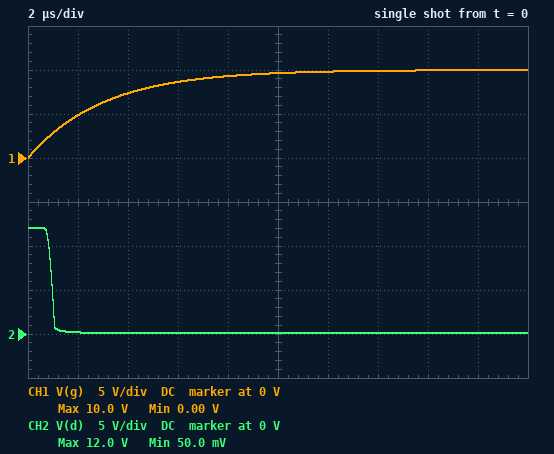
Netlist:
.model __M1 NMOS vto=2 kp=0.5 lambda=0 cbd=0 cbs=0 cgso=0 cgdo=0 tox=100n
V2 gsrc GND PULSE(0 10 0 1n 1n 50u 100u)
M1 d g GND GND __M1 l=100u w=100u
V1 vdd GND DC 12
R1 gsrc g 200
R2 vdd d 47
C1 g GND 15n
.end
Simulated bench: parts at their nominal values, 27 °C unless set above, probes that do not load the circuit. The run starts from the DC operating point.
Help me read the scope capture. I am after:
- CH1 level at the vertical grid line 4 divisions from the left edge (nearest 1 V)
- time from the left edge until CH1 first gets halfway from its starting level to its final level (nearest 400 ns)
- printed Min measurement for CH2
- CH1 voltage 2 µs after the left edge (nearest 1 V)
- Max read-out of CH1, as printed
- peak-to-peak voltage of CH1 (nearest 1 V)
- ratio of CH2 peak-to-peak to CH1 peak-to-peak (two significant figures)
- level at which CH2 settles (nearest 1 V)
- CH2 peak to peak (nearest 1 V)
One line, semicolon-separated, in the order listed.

9 V; 2.0 µs; 50.0 mV; 5 V; 10.0 V; 10 V; 1.2; 0 V; 12 V
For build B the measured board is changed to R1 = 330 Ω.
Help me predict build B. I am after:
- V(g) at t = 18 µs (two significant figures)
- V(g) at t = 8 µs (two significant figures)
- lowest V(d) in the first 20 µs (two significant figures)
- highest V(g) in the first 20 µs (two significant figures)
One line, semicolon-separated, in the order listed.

9.7 V; 8.0 V; 65 mV; 9.8 V
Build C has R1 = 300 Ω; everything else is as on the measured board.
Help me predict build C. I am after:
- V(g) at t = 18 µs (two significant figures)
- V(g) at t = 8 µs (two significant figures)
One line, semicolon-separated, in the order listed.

9.8 V; 8.3 V
